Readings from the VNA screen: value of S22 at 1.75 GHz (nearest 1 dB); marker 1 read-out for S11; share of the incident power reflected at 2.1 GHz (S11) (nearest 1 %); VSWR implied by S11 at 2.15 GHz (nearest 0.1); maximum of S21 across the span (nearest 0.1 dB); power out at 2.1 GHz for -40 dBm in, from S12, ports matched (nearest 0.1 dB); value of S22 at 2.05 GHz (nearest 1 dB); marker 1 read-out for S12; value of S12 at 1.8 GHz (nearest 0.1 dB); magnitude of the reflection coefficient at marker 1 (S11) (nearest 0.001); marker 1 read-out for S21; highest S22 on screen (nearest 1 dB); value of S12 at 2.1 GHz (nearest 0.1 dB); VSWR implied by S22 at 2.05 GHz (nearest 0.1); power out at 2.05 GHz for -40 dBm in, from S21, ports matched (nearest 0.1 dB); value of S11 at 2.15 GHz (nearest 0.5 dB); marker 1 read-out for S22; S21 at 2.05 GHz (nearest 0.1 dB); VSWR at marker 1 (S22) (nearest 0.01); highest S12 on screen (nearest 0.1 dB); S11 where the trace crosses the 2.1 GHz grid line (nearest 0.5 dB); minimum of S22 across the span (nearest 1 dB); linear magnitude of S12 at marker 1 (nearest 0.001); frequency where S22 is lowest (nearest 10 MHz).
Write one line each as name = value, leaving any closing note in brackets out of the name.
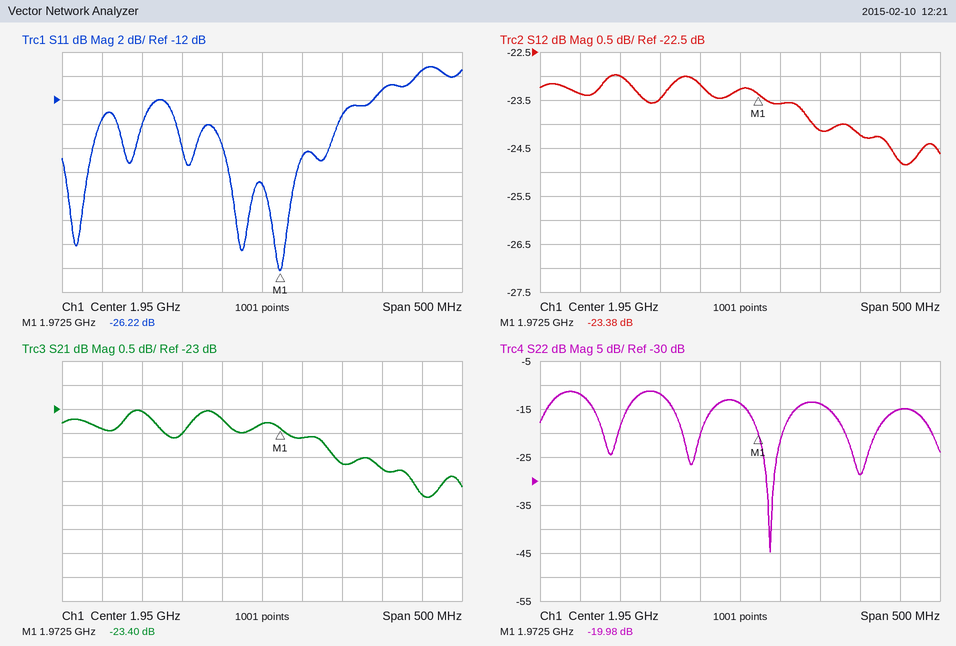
value of S22 at 1.75 GHz = -12 dB
marker 1 read-out for S11 = -26.22 dB
share of the incident power reflected at 2.1 GHz (S11) = 8 %
VSWR implied by S11 at 2.15 GHz = 2.0
maximum of S21 across the span = -23.0 dB
power out at 2.1 GHz for -40 dBm in, from S12, ports matched = -64.2 dBm
value of S22 at 2.05 GHz = -14 dB
marker 1 read-out for S12 = -23.38 dB
value of S12 at 1.8 GHz = -23.0 dB
magnitude of the reflection coefficient at marker 1 (S11) = 0.049
marker 1 read-out for S21 = -23.40 dB
highest S22 on screen = -11 dB
value of S12 at 2.1 GHz = -24.2 dB
VSWR implied by S22 at 2.05 GHz = 1.5
power out at 2.05 GHz for -40 dBm in, from S21, ports matched = -64.1 dBm
value of S11 at 2.15 GHz = -9.5 dB
marker 1 read-out for S22 = -19.98 dB
S21 at 2.05 GHz = -24.1 dB
VSWR at marker 1 (S22) = 1.22
highest S12 on screen = -23.0 dB
S11 where the trace crosses the 2.1 GHz grid line = -11.0 dB
minimum of S22 across the span = -45 dB
linear magnitude of S12 at marker 1 = 0.068
frequency where S22 is lowest = 1.99 GHz
